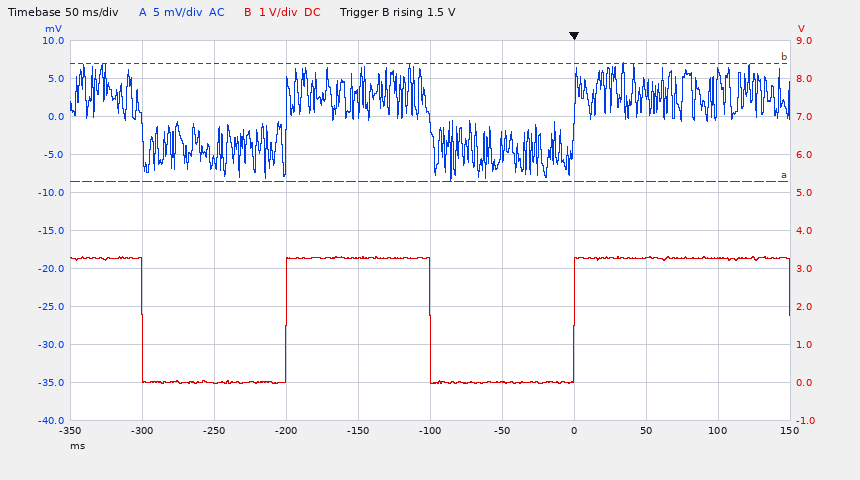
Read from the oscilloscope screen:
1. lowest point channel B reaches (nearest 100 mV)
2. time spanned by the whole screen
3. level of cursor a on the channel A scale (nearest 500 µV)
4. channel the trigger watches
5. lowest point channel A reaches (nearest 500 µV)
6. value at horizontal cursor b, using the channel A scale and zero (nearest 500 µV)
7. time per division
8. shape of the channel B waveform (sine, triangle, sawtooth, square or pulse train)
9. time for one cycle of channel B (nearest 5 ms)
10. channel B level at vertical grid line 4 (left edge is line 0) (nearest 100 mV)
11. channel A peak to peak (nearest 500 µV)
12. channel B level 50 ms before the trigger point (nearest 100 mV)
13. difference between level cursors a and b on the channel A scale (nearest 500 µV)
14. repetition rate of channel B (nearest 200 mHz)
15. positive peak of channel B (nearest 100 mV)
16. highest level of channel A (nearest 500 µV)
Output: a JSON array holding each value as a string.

["0.0 V", "500 ms", "-8.5 mV", "channel B", "-8.5 mV", "7.0 mV", "50 ms", "square", "200 ms", "3.3 V", "15.5 mV", "0.0 V", "15.5 mV", "5.0 Hz", "3.3 V", "7.0 mV"]
